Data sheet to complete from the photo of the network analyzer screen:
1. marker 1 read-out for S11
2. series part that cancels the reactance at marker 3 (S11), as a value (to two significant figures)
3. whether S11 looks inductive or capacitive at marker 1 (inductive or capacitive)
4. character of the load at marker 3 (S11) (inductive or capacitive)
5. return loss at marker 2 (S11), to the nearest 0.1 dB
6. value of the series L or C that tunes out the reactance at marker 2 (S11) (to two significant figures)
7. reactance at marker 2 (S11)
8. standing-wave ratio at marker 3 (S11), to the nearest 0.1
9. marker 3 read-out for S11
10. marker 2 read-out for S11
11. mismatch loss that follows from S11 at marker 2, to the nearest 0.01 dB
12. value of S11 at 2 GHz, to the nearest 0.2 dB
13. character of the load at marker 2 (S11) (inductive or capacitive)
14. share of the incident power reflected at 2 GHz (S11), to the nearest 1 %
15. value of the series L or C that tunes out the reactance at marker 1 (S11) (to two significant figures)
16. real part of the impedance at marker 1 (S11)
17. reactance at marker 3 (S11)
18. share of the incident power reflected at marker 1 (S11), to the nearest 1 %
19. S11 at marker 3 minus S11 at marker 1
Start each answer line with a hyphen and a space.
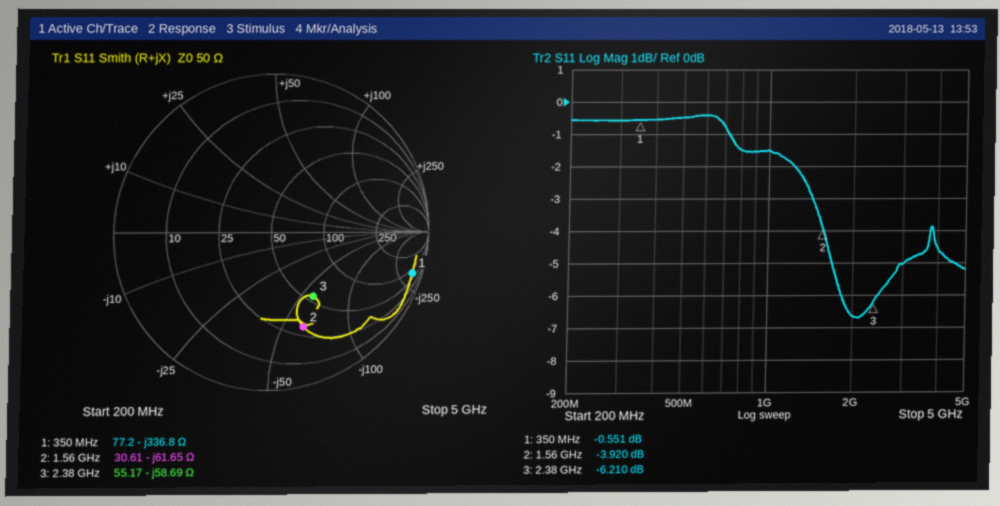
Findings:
- -0.551 dB
- 3.9 nH
- capacitive
- capacitive
- 3.9 dB
- 6.3 nH
- -61.65 Ω
- 2.9
- -6.210 dB
- -3.920 dB
- 2.26 dB
- -6.6 dB
- capacitive
- 22 %
- 150 nH
- 77.2 Ω
- -58.69 Ω
- 88 %
- -5.659 dB
